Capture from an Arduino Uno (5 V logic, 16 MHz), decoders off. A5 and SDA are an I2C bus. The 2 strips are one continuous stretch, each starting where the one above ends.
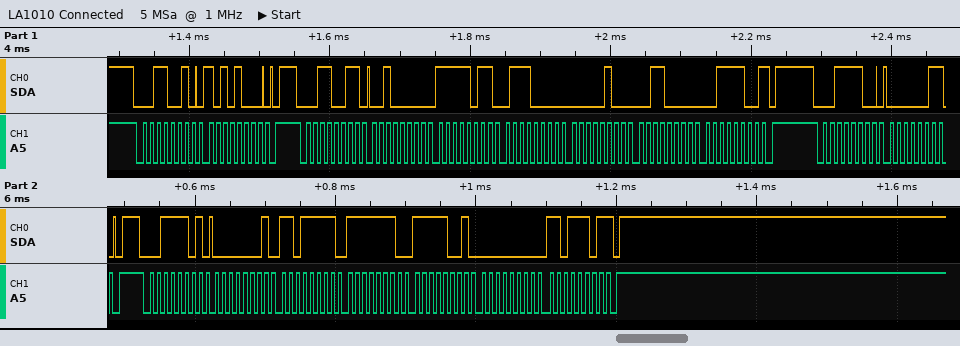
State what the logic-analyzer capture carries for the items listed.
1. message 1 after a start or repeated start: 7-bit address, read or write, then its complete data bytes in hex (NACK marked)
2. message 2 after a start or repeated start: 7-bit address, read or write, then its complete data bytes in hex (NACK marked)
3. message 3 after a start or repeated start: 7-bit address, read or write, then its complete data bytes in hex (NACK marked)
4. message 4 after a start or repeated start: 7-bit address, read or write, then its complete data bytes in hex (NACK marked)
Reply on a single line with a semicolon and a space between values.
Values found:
0x19 write: A8; 0x19 read: 20 FB 70 04 30 3C NACK; 0x1E write: 03; 0x1E read: 01 DF FE F9 00 DD NACK
